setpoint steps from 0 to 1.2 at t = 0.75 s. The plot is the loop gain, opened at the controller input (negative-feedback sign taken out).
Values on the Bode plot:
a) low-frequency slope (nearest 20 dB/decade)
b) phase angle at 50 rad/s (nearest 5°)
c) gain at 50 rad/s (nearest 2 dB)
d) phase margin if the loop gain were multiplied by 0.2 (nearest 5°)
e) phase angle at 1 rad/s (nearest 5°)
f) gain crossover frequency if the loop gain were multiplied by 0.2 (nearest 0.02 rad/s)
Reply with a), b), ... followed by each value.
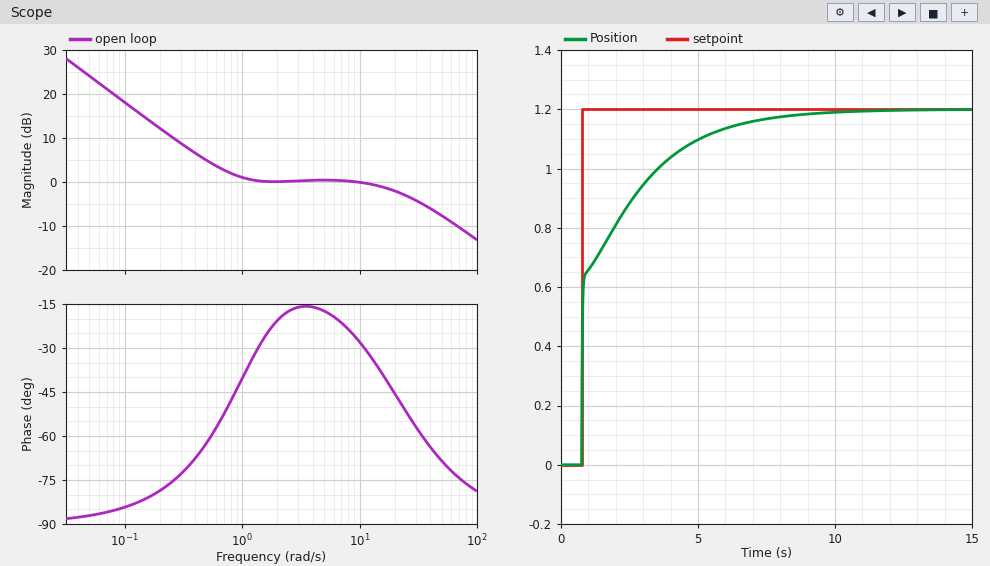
a) -20 dB/decade
b) -70°
c) -8 dB
d) 100°
e) -40°
f) 0.16 rad/s
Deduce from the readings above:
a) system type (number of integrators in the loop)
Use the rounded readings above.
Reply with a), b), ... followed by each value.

a) 1
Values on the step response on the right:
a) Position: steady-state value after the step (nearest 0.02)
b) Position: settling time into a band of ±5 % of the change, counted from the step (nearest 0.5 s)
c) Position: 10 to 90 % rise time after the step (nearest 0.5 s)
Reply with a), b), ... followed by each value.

a) 1.20
b) 5.5 s
c) 4.0 s
